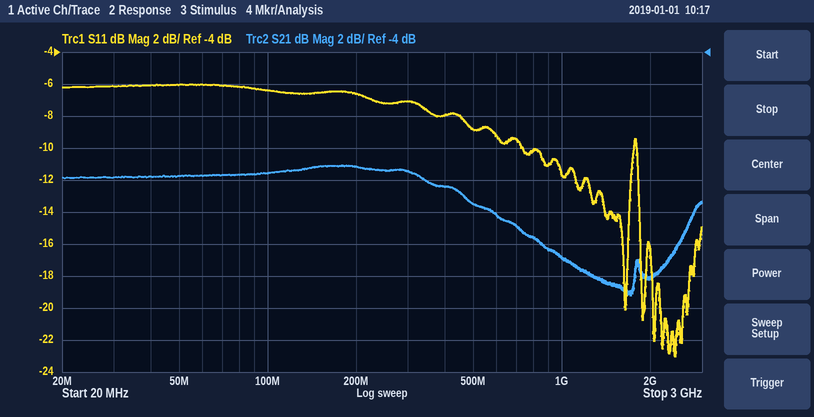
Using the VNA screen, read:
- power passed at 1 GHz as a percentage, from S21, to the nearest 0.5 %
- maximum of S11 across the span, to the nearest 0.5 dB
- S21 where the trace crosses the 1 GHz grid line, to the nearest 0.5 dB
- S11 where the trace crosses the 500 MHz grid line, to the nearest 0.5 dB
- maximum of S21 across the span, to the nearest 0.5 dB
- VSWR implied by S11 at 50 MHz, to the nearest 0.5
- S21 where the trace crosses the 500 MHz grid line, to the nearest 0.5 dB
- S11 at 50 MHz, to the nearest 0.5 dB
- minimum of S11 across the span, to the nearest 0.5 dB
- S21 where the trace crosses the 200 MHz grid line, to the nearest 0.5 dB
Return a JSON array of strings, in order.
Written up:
["2.0 %", "-6.0 dB", "-17.0 dB", "-9.0 dB", "-11.0 dB", "3.0", "-13.5 dB", "-6.0 dB", "-23.0 dB", "-11.0 dB"]
